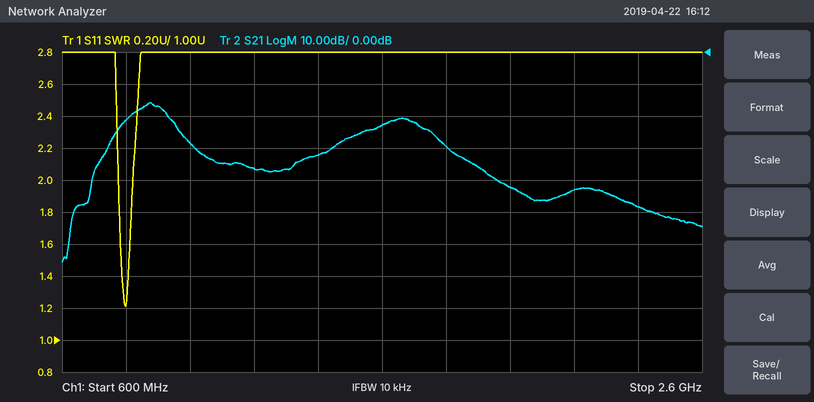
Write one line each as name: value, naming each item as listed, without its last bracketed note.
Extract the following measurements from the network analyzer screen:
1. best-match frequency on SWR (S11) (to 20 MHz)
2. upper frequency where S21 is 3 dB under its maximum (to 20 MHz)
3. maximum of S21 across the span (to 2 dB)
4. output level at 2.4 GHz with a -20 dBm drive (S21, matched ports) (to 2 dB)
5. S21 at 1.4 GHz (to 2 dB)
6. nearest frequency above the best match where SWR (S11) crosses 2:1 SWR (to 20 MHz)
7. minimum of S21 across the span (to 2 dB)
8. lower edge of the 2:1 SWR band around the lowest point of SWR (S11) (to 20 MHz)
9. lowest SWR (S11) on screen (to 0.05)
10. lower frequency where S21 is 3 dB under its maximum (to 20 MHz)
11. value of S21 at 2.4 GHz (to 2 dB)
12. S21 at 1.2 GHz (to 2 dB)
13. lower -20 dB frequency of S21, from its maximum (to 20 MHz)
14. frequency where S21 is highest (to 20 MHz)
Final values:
best-match frequency on SWR (S11): 800 MHz
upper frequency where S21 is 3 dB under its maximum: 920 MHz
maximum of S21 across the span: -16 dB
output level at 2.4 GHz with a -20 dBm drive (S21, matched ports): -68 dBm
S21 at 1.4 GHz: -32 dB
nearest frequency above the best match where SWR (S11) crosses 2:1 SWR: 820 MHz
minimum of S21 across the span: -66 dB
lower edge of the 2:1 SWR band around the lowest point of SWR (S11): 780 MHz
lowest SWR (S11) on screen: 1.20
lower frequency where S21 is 3 dB under its maximum: 820 MHz
value of S21 at 2.4 GHz: -48 dB
S21 at 1.2 GHz: -36 dB
lower -20 dB frequency of S21, from its maximum: 700 MHz
frequency where S21 is highest: 880 MHz
